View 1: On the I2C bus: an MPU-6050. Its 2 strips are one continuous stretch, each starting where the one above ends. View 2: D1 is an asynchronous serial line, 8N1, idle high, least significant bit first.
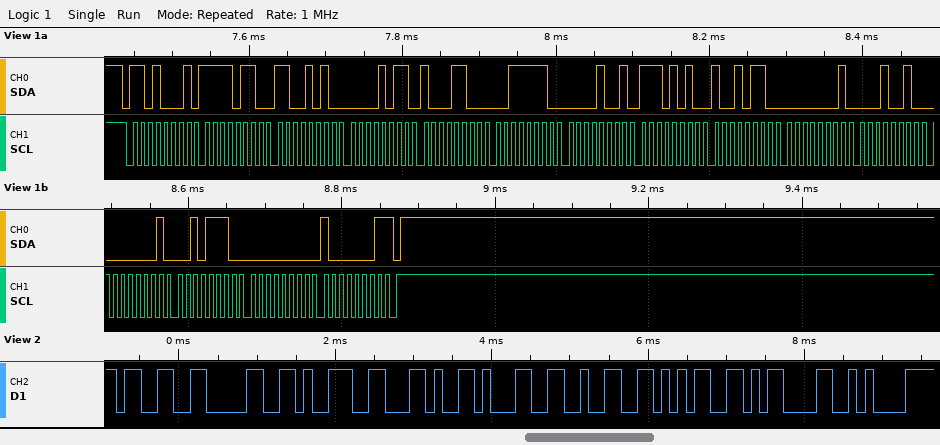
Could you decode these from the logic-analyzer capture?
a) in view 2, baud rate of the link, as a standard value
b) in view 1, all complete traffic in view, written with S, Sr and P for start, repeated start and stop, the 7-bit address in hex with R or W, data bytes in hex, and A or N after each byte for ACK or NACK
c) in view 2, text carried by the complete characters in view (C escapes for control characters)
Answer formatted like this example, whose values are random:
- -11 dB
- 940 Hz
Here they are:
- 9600 baud
- S 68R A F6 A CA A 0B A 8C A 3E A 09 A EA A 96 A 01 A 12 A 01 A 2E A 00 A 81 N P
- "309,125\r\n"
